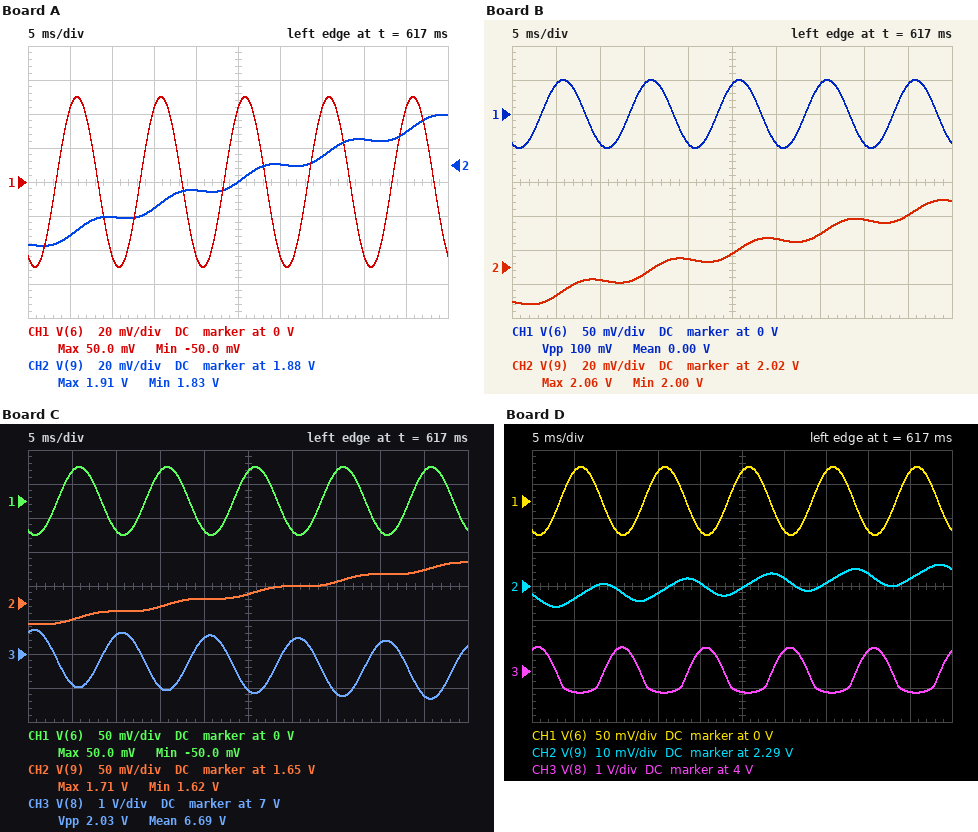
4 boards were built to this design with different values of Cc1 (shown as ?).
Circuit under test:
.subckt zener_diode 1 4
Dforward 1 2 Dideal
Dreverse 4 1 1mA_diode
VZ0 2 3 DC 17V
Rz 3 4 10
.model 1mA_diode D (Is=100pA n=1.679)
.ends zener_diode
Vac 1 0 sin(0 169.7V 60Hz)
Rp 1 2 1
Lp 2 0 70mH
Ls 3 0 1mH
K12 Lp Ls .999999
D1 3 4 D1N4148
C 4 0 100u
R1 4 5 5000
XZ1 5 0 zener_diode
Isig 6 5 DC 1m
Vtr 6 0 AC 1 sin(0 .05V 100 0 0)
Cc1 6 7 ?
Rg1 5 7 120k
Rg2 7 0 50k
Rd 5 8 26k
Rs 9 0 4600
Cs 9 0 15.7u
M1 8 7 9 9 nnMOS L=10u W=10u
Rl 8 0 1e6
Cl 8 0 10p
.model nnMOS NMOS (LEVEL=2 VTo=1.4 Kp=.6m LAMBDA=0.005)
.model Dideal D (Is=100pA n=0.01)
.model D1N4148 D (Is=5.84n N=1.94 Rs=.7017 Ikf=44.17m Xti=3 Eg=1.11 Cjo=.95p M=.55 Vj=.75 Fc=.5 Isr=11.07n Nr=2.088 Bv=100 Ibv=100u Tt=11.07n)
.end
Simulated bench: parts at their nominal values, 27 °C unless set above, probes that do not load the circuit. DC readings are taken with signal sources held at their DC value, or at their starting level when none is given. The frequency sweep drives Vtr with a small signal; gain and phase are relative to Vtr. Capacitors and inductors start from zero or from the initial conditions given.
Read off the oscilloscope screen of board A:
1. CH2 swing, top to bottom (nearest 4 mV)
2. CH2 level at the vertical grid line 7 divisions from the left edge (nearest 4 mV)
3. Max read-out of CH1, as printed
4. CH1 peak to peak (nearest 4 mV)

76 mV
1.884 V
50.0 mV
100 mV
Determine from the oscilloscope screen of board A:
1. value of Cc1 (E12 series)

8.2 µF
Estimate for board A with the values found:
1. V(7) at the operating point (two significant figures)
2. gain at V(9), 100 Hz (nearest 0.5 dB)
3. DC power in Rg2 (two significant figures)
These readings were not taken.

5.0 V
-22.5 dB
500 µW
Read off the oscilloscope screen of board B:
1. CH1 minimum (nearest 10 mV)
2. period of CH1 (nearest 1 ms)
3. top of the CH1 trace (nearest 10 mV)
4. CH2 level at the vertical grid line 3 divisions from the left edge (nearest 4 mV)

-50 mV
10 ms
50 mV
2.016 V
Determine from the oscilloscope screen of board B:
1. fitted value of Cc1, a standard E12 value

6.8 µF
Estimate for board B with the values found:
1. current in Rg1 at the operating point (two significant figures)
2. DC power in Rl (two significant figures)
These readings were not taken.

100 µA
15 µW
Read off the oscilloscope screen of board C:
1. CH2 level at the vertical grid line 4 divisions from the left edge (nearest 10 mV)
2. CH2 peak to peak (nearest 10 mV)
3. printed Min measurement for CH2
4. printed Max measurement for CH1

1.66 V
90 mV
1.62 V
50.0 mV
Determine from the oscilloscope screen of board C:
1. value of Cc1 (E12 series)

10 µF
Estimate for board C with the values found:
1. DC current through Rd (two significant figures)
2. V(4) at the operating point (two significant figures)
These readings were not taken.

510 µA
17 V
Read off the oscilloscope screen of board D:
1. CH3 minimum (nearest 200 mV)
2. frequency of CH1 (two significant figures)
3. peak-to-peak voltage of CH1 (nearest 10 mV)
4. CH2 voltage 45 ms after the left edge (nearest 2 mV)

3.4 V
100 Hz
100 mV
2.292 V
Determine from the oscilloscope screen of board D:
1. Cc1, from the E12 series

3.3 µF
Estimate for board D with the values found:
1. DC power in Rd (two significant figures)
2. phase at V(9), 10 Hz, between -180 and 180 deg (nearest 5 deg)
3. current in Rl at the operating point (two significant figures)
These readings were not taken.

6.7 mW
-40 deg
3.8 µA
